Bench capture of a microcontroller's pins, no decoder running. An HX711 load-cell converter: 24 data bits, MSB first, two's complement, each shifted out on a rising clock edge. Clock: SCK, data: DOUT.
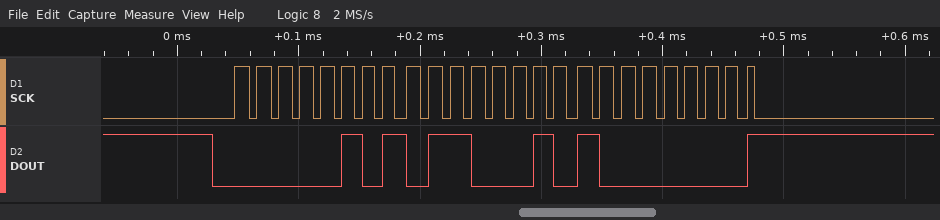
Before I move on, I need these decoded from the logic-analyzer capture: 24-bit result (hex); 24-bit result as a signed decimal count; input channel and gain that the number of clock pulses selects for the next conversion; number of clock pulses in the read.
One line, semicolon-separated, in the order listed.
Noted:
0x056280; 352896; channel A, gain 128; 25
